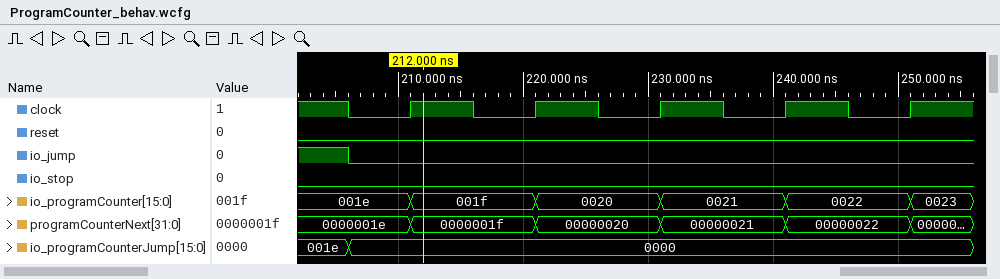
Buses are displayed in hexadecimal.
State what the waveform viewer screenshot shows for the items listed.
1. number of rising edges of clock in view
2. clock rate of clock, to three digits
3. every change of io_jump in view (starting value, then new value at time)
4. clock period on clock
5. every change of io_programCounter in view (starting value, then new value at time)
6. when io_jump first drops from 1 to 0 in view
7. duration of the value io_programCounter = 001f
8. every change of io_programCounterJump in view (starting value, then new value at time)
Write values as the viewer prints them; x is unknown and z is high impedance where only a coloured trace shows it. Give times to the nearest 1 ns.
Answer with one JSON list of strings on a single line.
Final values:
["5", "100 MHz", "1, 0 at 206 ns", "10 ns", "001e, 001f at 211 ns, 0020 at 221 ns, 0021 at 231 ns, 0022 at 241 ns, 0023 at 251 ns", "206 ns", "10 ns", "001e, 0000 at 206 ns"]
